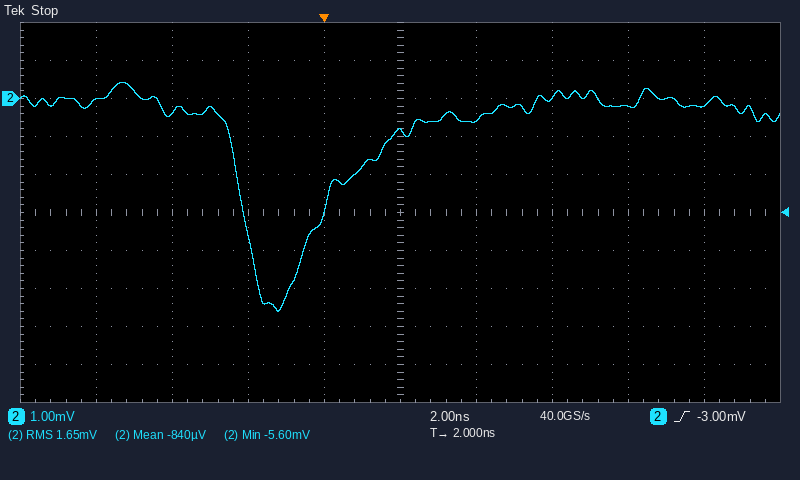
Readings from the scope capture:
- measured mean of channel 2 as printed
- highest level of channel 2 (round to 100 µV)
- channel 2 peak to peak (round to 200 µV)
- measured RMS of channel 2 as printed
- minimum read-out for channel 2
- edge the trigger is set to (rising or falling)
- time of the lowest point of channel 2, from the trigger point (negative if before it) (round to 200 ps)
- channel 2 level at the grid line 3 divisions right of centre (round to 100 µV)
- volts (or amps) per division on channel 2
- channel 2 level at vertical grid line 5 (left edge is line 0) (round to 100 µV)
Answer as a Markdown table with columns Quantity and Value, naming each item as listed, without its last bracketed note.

| Quantity | Value |
|---|---|
| measured mean of channel 2 as printed | -840 µV |
| highest level of channel 2 | 400 µV |
| channel 2 peak to peak | 6.0 mV |
| measured RMS of channel 2 as printed | 1.65 mV |
| minimum read-out for channel 2 | -5.60 mV |
| edge the trigger is set to | rising |
| time of the lowest point of channel 2, from the trigger point (negative if before it) | -1.2 ns |
| channel 2 level at the grid line 3 divisions right of centre | -200 µV |
| volts (or amps) per division on channel 2 | 1 mV |
| channel 2 level at vertical grid line 5 (left edge is line 0) | -900 µV |
